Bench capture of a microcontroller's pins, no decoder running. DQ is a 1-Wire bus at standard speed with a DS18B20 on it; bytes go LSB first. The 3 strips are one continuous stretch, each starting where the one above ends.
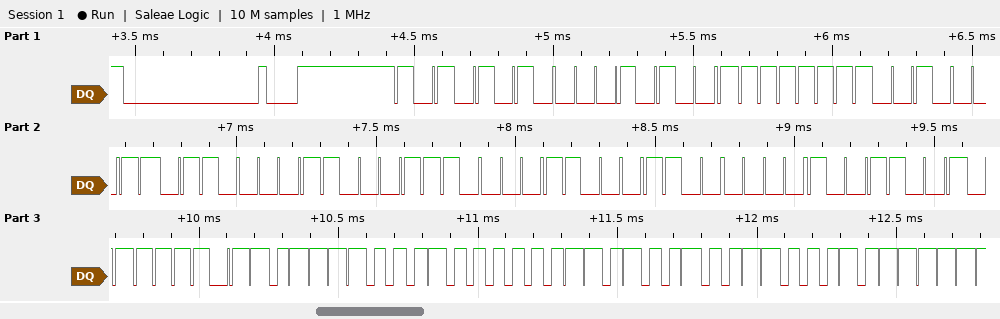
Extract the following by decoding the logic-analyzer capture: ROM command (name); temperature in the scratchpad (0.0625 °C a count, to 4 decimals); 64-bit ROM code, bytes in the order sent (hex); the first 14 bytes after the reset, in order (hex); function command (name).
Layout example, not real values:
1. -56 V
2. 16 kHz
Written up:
1. Match ROM
2. 35.8125 °C
3. 28 FF C4 86 71 18 03 99
4. 55 28 FF C4 86 71 18 03 99 BE 3D 02 4B 46
5. Read Scratchpad
